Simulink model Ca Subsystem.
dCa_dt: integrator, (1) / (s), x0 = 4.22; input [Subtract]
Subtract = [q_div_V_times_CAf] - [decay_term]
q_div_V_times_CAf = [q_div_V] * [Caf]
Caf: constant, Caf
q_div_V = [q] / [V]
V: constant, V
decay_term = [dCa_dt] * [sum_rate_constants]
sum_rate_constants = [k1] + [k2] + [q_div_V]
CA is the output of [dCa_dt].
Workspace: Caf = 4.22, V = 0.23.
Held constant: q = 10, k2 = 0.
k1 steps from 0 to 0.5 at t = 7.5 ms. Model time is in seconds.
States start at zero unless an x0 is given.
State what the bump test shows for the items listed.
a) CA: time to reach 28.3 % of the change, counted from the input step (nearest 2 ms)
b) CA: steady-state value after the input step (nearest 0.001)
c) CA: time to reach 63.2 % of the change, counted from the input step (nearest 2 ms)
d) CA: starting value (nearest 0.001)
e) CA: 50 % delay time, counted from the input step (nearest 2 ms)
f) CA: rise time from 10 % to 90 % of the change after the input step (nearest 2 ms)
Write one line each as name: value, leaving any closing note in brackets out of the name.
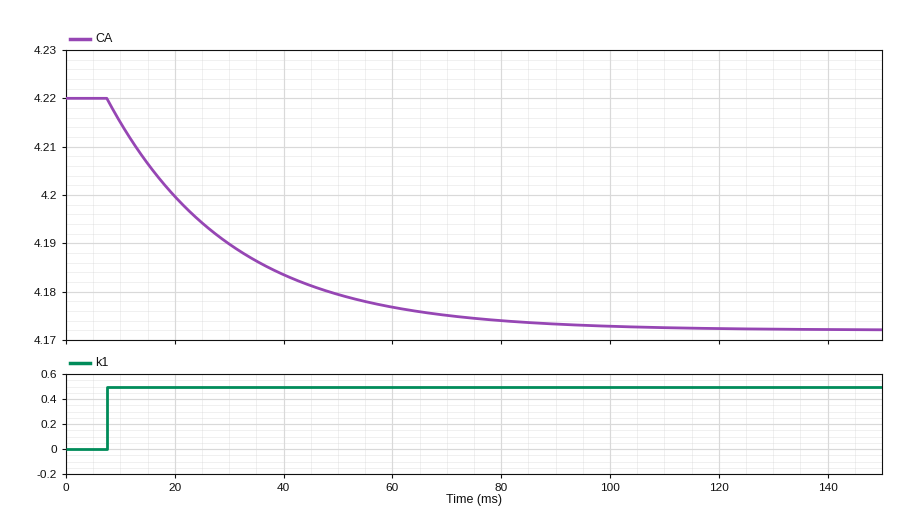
CA: time to reach 28.3 % of the change, counted from the input step: 8 ms
CA: steady-state value after the input step: 4.172
CA: time to reach 63.2 % of the change, counted from the input step: 22 ms
CA: starting value: 4.220
CA: 50 % delay time, counted from the input step: 16 ms
CA: rise time from 10 % to 90 % of the change after the input step: 50 ms
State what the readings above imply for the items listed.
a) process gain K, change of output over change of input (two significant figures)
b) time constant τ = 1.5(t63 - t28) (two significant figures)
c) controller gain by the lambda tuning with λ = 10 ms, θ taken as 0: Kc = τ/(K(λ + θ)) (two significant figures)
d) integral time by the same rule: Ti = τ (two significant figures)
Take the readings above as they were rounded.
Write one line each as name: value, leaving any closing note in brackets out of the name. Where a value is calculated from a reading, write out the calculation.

process gain K, change of output over change of input: (4.172 - 4.22) / 0.5 = -0.096
time constant τ = 1.5(t63 - t28): 1.5 × (22 - 8) = 21 ms
controller gain by the lambda tuning with λ = 10 ms, θ taken as 0: Kc = τ/(K(λ + θ)): 21 / (-0.096 × (10 + 0)) = -22
integral time by the same rule: Ti = τ: 21 ms
